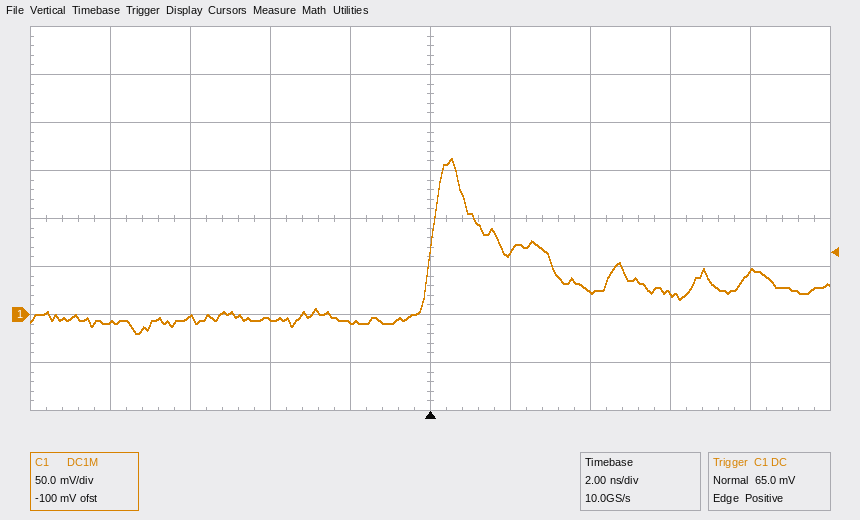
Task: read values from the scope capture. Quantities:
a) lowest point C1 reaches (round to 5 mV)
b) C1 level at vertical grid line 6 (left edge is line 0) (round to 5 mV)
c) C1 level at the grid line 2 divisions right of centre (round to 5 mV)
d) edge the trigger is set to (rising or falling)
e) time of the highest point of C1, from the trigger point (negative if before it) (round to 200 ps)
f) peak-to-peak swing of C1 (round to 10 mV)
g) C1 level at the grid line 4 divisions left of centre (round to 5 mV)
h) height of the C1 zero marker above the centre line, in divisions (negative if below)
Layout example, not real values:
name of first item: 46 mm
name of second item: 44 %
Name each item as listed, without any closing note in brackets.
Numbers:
lowest point C1 reaches: -20 mV
C1 level at vertical grid line 6 (left edge is line 0): 65 mV
C1 level at the grid line 2 divisions right of centre: 25 mV
edge the trigger is set to: rising
time of the highest point of C1, from the trigger point (negative if before it): +600 ps
peak-to-peak swing of C1: 180 mV
C1 level at the grid line 4 divisions left of centre: -10 mV
height of the C1 zero marker above the centre line, in divisions: -2.0 div
